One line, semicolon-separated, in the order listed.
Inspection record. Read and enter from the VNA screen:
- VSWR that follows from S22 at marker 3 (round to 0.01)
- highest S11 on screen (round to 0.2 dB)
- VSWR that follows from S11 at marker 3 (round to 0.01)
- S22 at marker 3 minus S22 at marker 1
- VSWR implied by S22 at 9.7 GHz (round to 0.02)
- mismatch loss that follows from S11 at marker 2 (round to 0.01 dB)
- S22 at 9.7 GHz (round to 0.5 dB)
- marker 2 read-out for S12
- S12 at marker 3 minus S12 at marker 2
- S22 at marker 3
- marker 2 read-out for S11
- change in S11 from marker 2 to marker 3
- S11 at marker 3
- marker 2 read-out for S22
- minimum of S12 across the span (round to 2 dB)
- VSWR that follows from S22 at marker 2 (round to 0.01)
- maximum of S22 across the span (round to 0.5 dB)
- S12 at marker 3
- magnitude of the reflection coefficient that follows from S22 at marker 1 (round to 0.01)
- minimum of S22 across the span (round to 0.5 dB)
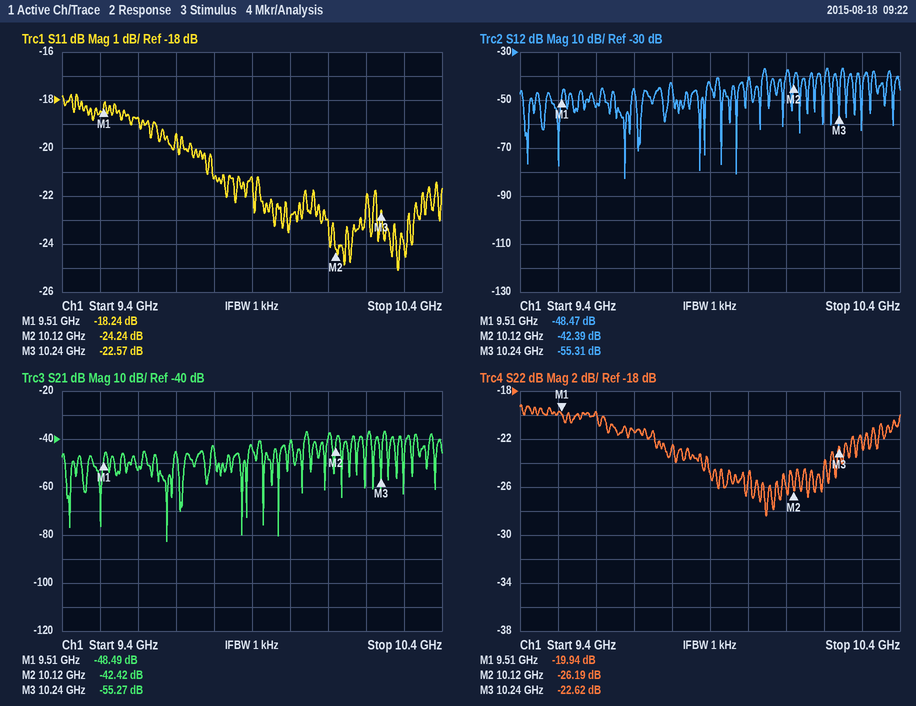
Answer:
1.16; -17.8 dB; 1.16; -2.68 dB; 1.18; 0.02 dB; -21.5 dB; -42.39 dB; -12.92 dB; -22.62 dB; -24.24 dB; 1.67 dB; -22.57 dB; -26.19 dB; -82 dB; 1.10; -19.0 dB; -55.31 dB; 0.10; -28.5 dB
